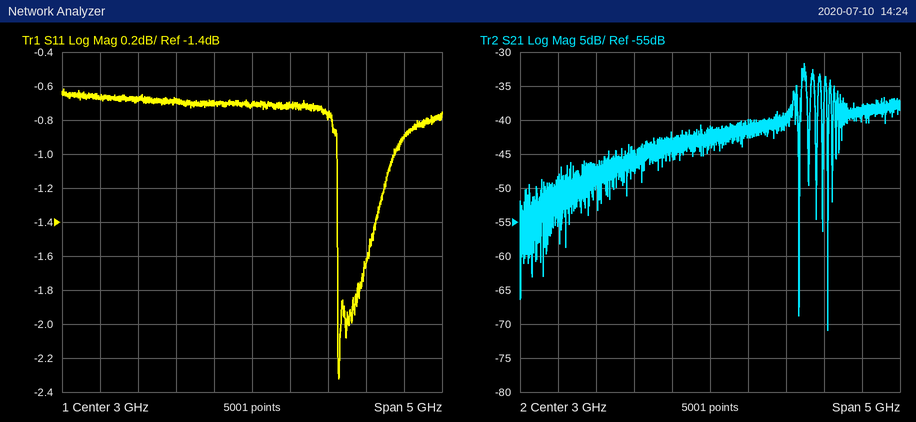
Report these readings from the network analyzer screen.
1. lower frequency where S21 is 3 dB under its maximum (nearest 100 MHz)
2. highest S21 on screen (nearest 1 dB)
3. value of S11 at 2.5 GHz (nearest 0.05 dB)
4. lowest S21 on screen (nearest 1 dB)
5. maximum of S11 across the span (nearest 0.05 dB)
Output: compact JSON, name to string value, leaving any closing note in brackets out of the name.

{"lower frequency where S21 is 3 dB under its maximum": "4.2 GHz", "highest S21 on screen": "-32 dB", "value of S11 at 2.5 GHz": "-0.70 dB", "lowest S21 on screen": "-71 dB", "maximum of S11 across the span": "-0.60 dB"}
